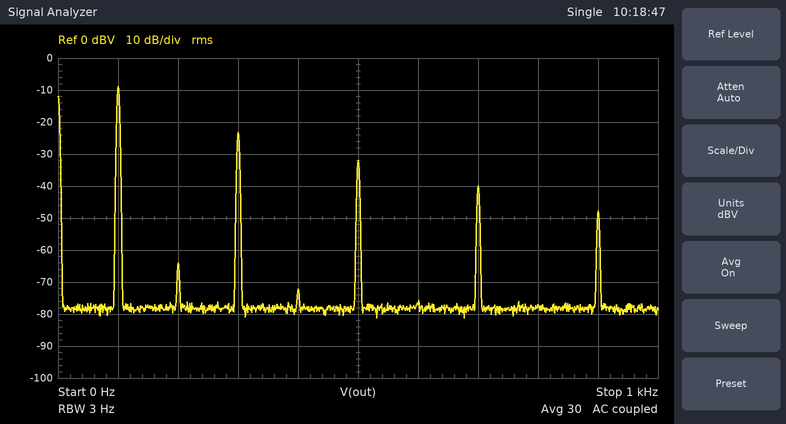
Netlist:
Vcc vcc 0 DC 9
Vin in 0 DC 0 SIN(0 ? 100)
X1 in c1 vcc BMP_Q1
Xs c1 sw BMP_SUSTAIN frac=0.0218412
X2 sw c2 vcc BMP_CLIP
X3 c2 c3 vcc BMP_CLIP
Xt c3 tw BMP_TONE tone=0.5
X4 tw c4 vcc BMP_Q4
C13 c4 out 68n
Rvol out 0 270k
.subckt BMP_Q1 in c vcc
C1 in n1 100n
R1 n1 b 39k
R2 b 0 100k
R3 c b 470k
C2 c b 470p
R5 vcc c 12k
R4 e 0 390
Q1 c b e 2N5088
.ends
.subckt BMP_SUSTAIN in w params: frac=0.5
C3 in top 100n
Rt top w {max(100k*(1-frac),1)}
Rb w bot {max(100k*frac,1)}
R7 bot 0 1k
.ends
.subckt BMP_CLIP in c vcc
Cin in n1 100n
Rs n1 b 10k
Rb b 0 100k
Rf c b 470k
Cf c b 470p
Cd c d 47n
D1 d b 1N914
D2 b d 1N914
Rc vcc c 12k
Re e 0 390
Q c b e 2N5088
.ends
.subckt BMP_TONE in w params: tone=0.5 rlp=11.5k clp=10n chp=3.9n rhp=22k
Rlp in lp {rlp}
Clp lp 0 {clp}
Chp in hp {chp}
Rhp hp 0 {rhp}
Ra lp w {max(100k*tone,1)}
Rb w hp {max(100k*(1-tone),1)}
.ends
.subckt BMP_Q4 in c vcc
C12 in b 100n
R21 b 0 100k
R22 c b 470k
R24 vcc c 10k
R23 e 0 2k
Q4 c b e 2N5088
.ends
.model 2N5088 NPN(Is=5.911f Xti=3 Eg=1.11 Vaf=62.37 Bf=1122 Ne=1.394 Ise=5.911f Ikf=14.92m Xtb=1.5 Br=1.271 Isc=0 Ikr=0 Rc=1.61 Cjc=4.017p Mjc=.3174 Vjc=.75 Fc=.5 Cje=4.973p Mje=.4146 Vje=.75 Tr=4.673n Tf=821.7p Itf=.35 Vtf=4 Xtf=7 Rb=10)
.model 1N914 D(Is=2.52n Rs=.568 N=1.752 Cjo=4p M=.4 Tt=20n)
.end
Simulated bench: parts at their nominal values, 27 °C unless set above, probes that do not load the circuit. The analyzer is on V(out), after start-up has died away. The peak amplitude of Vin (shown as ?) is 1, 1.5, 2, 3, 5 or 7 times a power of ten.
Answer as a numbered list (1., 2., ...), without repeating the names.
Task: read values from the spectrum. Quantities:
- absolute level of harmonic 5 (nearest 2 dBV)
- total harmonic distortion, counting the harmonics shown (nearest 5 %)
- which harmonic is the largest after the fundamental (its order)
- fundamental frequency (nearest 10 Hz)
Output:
1. -32 dBV
2. 20 %
3. 3
4. 100 Hz
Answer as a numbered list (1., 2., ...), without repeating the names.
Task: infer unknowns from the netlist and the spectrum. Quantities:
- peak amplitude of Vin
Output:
1. 50 mV
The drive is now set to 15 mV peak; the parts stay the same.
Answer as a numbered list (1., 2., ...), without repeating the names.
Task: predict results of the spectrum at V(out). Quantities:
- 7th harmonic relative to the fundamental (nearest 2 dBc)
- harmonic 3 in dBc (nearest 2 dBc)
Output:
1. -54 dBc
2. -22 dBc
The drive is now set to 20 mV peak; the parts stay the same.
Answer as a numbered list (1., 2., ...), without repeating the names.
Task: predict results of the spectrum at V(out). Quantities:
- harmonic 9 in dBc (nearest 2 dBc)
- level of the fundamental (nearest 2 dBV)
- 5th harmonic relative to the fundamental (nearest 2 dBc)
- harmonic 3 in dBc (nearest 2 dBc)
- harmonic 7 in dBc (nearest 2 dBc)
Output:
1. -56 dBc
2. -12 dBV
3. -36 dBc
4. -20 dBc
5. -50 dBc
